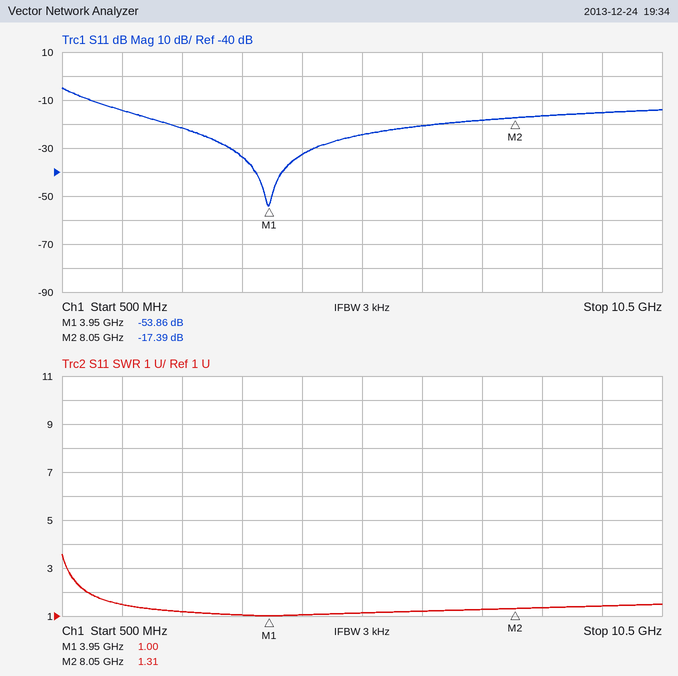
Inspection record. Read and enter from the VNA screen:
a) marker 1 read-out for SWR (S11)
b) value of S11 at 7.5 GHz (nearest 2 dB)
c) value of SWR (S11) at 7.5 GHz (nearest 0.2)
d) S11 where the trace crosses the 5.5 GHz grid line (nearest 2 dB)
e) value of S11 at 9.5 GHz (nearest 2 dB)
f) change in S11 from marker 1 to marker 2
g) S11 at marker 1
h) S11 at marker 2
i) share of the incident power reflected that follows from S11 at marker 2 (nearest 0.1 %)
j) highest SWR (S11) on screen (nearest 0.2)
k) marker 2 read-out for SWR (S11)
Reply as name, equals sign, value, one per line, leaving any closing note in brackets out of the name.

marker 1 read-out for SWR = 1.00
value of S11 at 7.5 GHz = -18 dB
value of SWR (S11) at 7.5 GHz = 1.2
S11 where the trace crosses the 5.5 GHz grid line = -24 dB
value of S11 at 9.5 GHz = -16 dB
change in S11 from marker 1 to marker 2 = 36.47 dB
S11 at marker 1 = -53.86 dB
S11 at marker 2 = -17.39 dB
share of the incident power reflected that follows from S11 at marker 2 = 1.8 %
highest SWR (S11) on screen = 3.6
marker 2 read-out for SWR = 1.31
